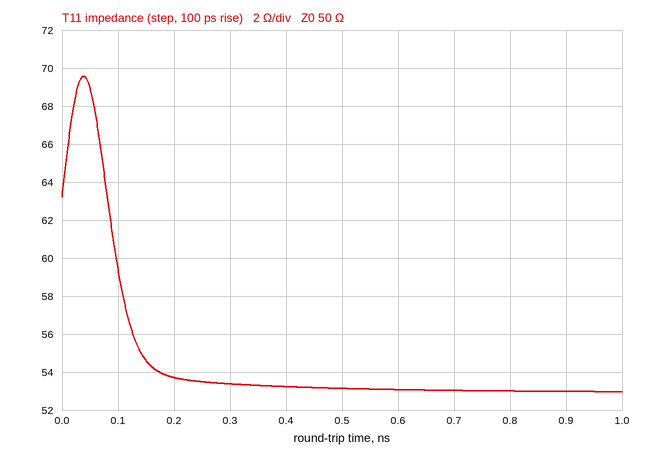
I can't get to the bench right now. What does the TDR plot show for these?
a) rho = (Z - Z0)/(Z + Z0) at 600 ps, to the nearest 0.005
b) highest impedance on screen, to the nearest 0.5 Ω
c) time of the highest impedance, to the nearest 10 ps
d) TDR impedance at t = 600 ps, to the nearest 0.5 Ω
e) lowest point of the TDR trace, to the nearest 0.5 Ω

+0.030
69.5 Ω
40 ps
53.0 Ω
53.0 Ω
